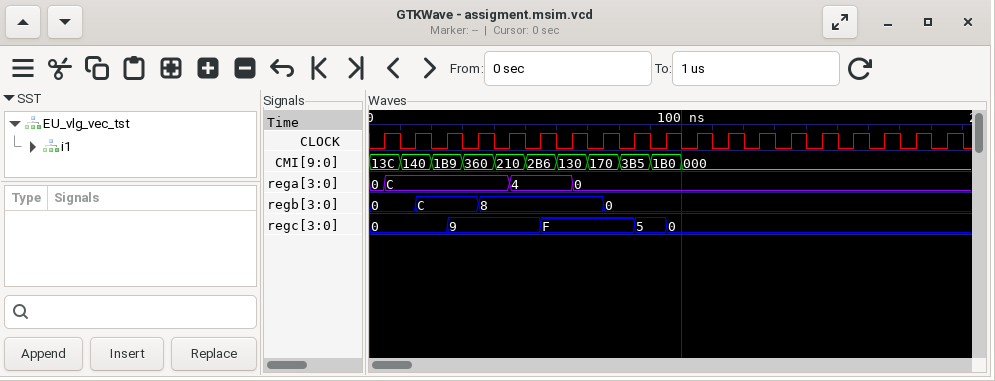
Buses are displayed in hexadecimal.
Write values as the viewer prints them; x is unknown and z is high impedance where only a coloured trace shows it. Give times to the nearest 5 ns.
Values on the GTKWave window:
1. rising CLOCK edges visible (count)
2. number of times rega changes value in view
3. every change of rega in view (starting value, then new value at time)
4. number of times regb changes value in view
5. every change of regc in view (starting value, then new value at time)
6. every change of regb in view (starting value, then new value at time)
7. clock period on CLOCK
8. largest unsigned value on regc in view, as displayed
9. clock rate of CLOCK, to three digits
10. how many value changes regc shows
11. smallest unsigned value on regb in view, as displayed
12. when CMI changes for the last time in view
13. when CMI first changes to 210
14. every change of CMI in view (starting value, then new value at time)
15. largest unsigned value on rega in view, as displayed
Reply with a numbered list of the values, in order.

1. 19
2. 3
3. 0, C at 5 ns, 4 at 45 ns, 0 at 65 ns
4. 3
5. 0, 9 at 25 ns, F at 55 ns, 5 at 85 ns, 0 at 95 ns
6. 0, C at 15 ns, 8 at 35 ns, 0 at 75 ns
7. 10 ns
8. F
9. 100 MHz
10. 4
11. 0
12. 100 ns
13. 40 ns
14. 13C, 140 at 10 ns, 1B9 at 20 ns, 360 at 30 ns, 210 at 40 ns, 2B6 at 50 ns, 130 at 60 ns, 170 at 70 ns, 3B5 at 80 ns, 1B0 at 90 ns, 000 at 100 ns
15. C
